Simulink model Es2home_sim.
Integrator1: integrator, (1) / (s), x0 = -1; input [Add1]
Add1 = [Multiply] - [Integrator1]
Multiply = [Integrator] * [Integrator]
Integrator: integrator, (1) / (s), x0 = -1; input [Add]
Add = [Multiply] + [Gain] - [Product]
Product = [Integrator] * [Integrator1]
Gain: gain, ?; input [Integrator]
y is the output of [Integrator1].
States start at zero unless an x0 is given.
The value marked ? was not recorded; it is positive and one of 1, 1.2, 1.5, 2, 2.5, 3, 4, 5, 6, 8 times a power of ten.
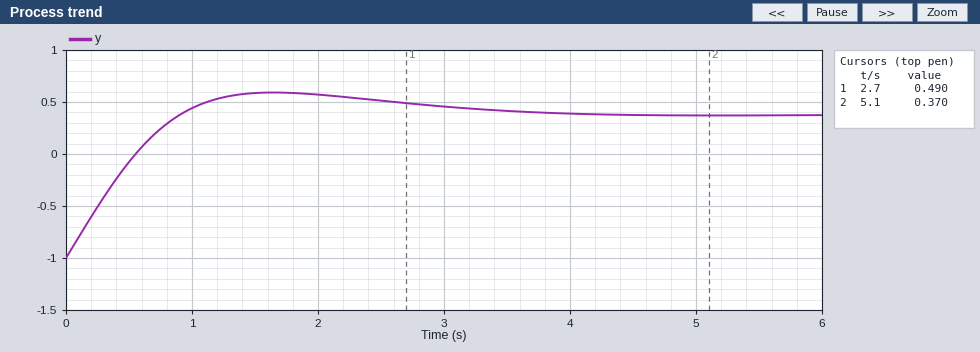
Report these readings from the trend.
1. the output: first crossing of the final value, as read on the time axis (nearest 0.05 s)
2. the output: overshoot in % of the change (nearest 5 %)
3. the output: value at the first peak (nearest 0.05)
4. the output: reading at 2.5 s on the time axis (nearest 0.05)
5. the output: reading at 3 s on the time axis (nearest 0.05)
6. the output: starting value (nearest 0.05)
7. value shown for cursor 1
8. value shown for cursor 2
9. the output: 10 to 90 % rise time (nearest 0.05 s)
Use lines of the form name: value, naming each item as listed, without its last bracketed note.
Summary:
the output: first crossing of the final value, as read on the time axis: 0.90 s
the output: overshoot in % of the change: 15 %
the output: value at the first peak: 0.60
the output: reading at 2.5 s on the time axis: 0.50
the output: reading at 3 s on the time axis: 0.45
the output: starting value: -1.00
value shown for cursor 1: 0.490
value shown for cursor 2: 0.370
the output: 10 to 90 % rise time: 0.70 s
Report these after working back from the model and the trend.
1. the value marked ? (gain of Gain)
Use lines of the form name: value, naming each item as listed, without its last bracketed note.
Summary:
the value marked ?: 1
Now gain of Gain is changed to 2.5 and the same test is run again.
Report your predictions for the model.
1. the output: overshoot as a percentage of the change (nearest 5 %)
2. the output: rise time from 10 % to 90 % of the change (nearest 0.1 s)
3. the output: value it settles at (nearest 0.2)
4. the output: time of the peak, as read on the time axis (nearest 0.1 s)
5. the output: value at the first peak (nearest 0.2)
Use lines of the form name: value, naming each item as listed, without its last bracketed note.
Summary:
the output: overshoot as a percentage of the change: 15 %
the output: rise time from 10 % to 90 % of the change: 0.6 s
the output: value it settles at: 1.4
the output: time of the peak, as read on the time axis: 1.4 s
the output: value at the first peak: 1.6
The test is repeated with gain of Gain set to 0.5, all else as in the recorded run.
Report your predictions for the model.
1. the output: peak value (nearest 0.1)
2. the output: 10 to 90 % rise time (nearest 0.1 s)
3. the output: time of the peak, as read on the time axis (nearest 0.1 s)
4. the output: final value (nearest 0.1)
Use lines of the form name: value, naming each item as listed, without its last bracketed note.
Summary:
the output: peak value: 0.3
the output: 10 to 90 % rise time: 0.6 s
the output: time of the peak, as read on the time axis: 1.7 s
the output: final value: 0.1
